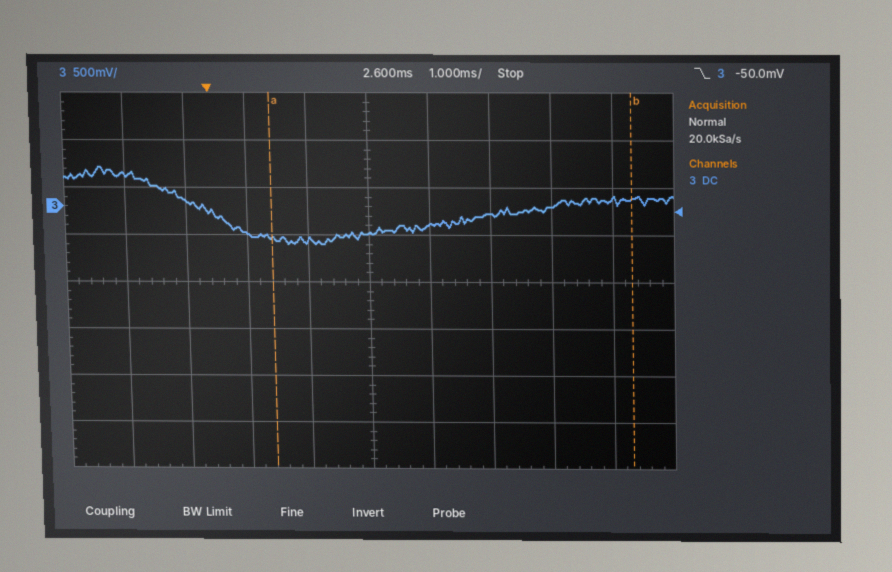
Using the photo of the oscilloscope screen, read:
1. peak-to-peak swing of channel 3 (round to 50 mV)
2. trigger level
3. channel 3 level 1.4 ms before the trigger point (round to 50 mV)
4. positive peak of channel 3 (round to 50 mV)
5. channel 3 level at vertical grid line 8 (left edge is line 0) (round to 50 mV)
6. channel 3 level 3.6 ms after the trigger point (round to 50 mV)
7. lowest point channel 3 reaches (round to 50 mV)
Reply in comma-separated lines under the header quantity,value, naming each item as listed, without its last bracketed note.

quantity,value
peak-to-peak swing of channel 3,800 mV
trigger level,-50.0 mV
channel 3 level 1.4 ms before the trigger point,350 mV
positive peak of channel 3,400 mV
channel 3 level at vertical grid line 8 (left edge is line 0),0 mV
channel 3 level 3.6 ms after the trigger point,-200 mV
lowest point channel 3 reaches,-400 mV
